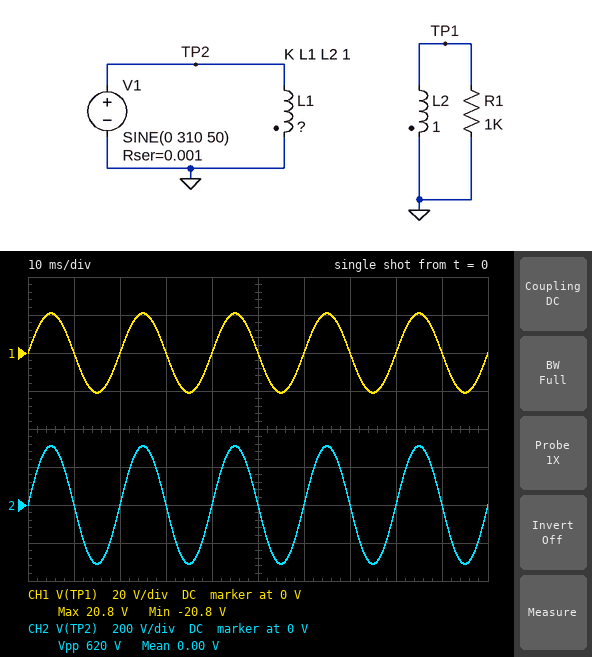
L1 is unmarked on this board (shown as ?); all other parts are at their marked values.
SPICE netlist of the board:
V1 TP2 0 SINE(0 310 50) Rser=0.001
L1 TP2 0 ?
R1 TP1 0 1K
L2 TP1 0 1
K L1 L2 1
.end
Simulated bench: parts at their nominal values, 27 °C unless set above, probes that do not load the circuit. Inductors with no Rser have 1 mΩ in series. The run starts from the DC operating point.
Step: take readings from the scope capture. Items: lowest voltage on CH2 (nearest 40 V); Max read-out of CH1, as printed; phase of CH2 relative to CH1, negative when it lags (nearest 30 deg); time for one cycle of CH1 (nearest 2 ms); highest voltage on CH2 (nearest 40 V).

-320 V
20.8 V
0 deg
20 ms
320 V
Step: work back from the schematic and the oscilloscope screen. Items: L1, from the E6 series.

220 H
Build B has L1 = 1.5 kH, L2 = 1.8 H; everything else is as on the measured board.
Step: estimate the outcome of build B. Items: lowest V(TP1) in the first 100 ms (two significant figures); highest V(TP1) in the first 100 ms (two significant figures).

-11 V
11 V
